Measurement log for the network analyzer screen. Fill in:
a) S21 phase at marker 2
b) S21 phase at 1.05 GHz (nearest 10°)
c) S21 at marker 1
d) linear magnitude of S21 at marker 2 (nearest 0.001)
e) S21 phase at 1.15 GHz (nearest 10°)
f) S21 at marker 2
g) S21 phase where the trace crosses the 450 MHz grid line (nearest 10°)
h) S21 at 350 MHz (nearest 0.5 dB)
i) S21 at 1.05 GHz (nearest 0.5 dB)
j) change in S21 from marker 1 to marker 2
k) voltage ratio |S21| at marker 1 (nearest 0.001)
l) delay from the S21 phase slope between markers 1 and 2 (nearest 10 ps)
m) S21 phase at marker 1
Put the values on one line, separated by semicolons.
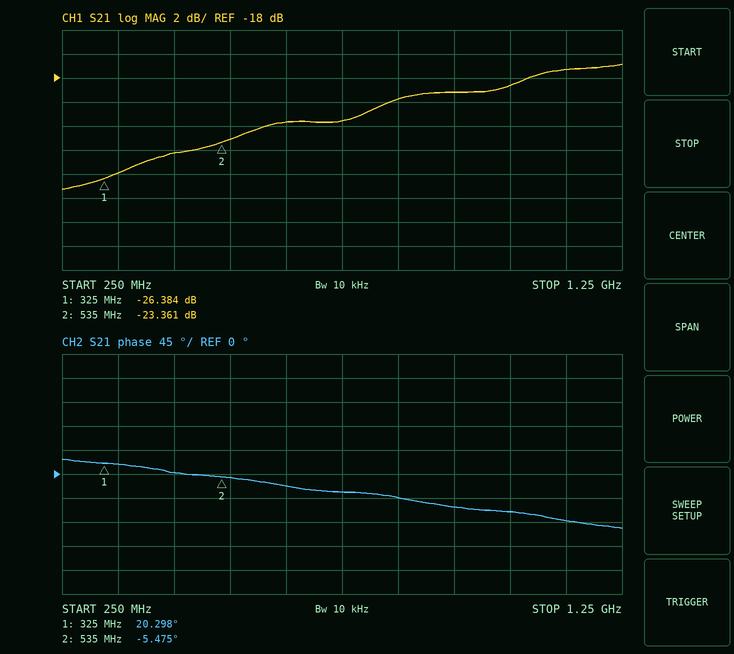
-5.475°; -70°; -26.384 dB; 0.068; -90°; -23.361 dB; 0°; -26.0 dB; -18.5 dB; 3.023 dB; 0.048; 340 ps; 20.298°
